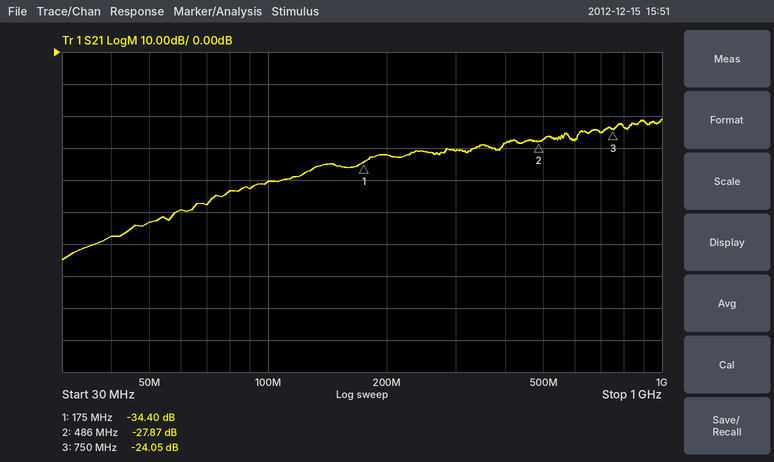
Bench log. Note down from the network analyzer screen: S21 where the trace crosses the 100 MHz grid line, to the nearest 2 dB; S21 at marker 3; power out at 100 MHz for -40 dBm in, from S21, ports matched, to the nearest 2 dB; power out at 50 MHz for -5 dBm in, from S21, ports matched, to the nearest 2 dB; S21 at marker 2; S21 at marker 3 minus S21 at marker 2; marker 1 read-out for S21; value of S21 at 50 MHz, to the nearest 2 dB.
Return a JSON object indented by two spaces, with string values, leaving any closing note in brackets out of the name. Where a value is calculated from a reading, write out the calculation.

{
  "S21 where the trace crosses the 100 MHz grid line, to the nearest 2 dB": "-40 dB",
  "S21 at marker 3": "-24.05 dB",
  "power out at 100 MHz for -40 dBm in, from S21, ports matched, to the nearest 2 dB": "-40 dBm + (-40 dB) = -80 dBm",
  "power out at 50 MHz for -5 dBm in, from S21, ports matched, to the nearest 2 dB": "-5 dBm + (-54 dB) = -58 dBm",
  "S21 at marker 2": "-27.87 dB",
  "S21 at marker 3 minus S21 at marker 2": "-24.05 − (-27.87) = 3.82 dB",
  "marker 1 read-out for S21": "-34.40 dB",
  "value of S21 at 50 MHz, to the nearest 2 dB": "-54 dB"
}
